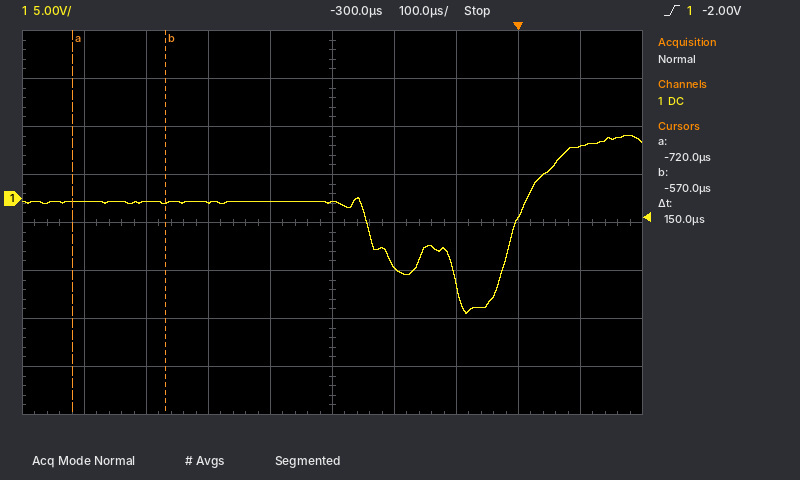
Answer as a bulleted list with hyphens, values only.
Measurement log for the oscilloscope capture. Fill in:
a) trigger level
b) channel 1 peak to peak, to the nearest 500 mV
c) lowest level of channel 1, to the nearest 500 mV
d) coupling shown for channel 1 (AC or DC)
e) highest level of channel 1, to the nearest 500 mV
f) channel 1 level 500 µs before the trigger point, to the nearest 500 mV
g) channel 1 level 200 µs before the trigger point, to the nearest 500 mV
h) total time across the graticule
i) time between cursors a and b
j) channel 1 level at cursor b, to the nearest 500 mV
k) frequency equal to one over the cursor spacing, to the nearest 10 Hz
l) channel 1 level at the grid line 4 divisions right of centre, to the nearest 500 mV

- -2.00 V
- 18.5 V
- -12.0 V
- DC
- 6.5 V
- -500 mV
- -7.0 V
- 1 ms
- 150 µs
- -500 mV
- 6.67 kHz
- 5.5 V
